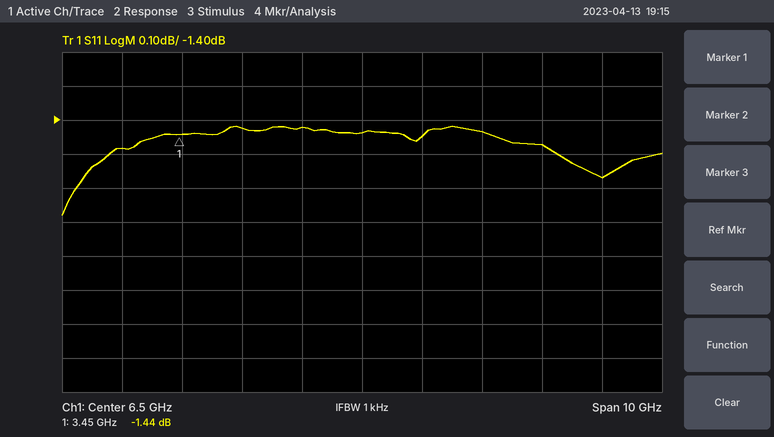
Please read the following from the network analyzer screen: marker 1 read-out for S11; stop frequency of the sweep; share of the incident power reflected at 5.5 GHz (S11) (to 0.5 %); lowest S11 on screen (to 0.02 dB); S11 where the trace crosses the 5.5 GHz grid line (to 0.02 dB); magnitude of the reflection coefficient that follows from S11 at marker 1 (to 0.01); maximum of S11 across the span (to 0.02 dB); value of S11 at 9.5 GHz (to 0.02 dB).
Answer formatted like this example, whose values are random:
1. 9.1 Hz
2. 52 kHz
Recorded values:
1. -1.44 dB
2. 11.5 GHz
3. 72.0 %
4. -1.68 dB
5. -1.42 dB
6. 0.85
7. -1.42 dB
8. -1.48 dB
